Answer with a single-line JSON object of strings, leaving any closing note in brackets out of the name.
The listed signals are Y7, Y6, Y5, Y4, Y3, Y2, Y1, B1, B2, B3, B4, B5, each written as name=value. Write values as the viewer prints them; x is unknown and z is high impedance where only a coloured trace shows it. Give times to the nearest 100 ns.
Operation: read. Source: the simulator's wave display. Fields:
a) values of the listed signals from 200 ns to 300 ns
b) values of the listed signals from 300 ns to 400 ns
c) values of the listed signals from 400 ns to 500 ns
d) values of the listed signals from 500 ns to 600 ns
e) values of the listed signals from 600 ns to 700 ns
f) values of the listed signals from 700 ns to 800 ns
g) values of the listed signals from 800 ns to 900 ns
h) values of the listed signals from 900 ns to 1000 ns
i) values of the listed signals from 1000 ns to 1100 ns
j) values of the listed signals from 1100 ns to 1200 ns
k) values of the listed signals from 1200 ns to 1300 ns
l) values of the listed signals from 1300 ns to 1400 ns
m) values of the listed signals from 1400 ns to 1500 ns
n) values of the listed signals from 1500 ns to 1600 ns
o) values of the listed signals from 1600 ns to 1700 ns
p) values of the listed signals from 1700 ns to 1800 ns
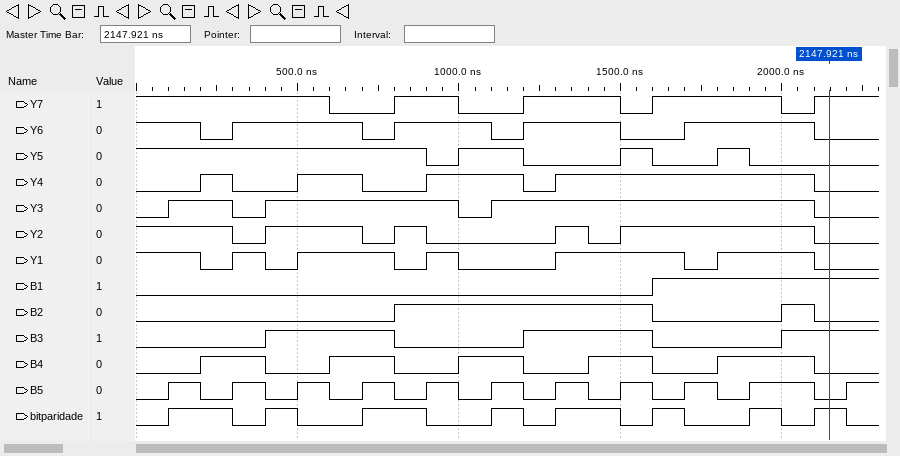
{"values of the listed signals from 200 ns to 300 ns": "Y7=1, Y6=0, Y5=1, Y4=1, Y3=1, Y2=1, Y1=0, B1=0, B2=0, B3=0, B4=1, B5=0", "values of the listed signals from 300 ns to 400 ns": "Y7=1, Y6=1, Y5=1, Y4=0, Y3=0, Y2=0, Y1=1, B1=0, B2=0, B3=0, B4=1, B5=1", "values of the listed signals from 400 ns to 500 ns": "Y7=1, Y6=1, Y5=1, Y4=0, Y3=1, Y2=1, Y1=0, B1=0, B2=0, B3=1, B4=0, B5=0", "values of the listed signals from 500 ns to 600 ns": "Y7=1, Y6=1, Y5=1, Y4=1, Y3=1, Y2=1, Y1=1, B1=0, B2=0, B3=1, B4=0, B5=1", "values of the listed signals from 600 ns to 700 ns": "Y7=0, Y6=1, Y5=1, Y4=1, Y3=1, Y2=1, Y1=1, B1=0, B2=0, B3=1, B4=1, B5=0", "values of the listed signals from 700 ns to 800 ns": "Y7=0, Y6=0, Y5=1, Y4=0, Y3=1, Y2=0, Y1=1, B1=0, B2=0, B3=1, B4=1, B5=1", "values of the listed signals from 800 ns to 900 ns": "Y7=1, Y6=1, Y5=1, Y4=0, Y3=1, Y2=1, Y1=0, B1=0, B2=1, B3=0, B4=0, B5=0", "values of the listed signals from 900 ns to 1000 ns": "Y7=1, Y6=1, Y5=0, Y4=1, Y3=1, Y2=0, Y1=1, B1=0, B2=1, B3=0, B4=0, B5=1", "values of the listed signals from 1000 ns to 1100 ns": "Y7=0, Y6=1, Y5=1, Y4=1, Y3=0, Y2=0, Y1=0, B1=0, B2=1, B3=0, B4=1, B5=0", "values of the listed signals from 1100 ns to 1200 ns": "Y7=0, Y6=0, Y5=1, Y4=1, Y3=1, Y2=0, Y1=0, B1=0, B2=1, B3=0, B4=1, B5=1", "values of the listed signals from 1200 ns to 1300 ns": "Y7=1, Y6=1, Y5=0, Y4=0, Y3=1, Y2=0, Y1=0, B1=0, B2=1, B3=1, B4=0, B5=0", "values of the listed signals from 1300 ns to 1400 ns": "Y7=1, Y6=1, Y5=0, Y4=1, Y3=1, Y2=1, Y1=1, B1=0, B2=1, B3=1, B4=0, B5=1", "values of the listed signals from 1400 ns to 1500 ns": "Y7=1, Y6=1, Y5=0, Y4=1, Y3=1, Y2=0, Y1=1, B1=0, B2=1, B3=1, B4=1, B5=0", "values of the listed signals from 1500 ns to 1600 ns": "Y7=0, Y6=0, Y5=1, Y4=1, Y3=1, Y2=1, Y1=1, B1=0, B2=1, B3=1, B4=1, B5=1", "values of the listed signals from 1600 ns to 1700 ns": "Y7=1, Y6=0, Y5=0, Y4=1, Y3=1, Y2=1, Y1=1, B1=1, B2=0, B3=0, B4=0, B5=0", "values of the listed signals from 1700 ns to 1800 ns": "Y7=1, Y6=1, Y5=0, Y4=1, Y3=1, Y2=1, Y1=0, B1=1, B2=0, B3=0, B4=0, B5=1"}
